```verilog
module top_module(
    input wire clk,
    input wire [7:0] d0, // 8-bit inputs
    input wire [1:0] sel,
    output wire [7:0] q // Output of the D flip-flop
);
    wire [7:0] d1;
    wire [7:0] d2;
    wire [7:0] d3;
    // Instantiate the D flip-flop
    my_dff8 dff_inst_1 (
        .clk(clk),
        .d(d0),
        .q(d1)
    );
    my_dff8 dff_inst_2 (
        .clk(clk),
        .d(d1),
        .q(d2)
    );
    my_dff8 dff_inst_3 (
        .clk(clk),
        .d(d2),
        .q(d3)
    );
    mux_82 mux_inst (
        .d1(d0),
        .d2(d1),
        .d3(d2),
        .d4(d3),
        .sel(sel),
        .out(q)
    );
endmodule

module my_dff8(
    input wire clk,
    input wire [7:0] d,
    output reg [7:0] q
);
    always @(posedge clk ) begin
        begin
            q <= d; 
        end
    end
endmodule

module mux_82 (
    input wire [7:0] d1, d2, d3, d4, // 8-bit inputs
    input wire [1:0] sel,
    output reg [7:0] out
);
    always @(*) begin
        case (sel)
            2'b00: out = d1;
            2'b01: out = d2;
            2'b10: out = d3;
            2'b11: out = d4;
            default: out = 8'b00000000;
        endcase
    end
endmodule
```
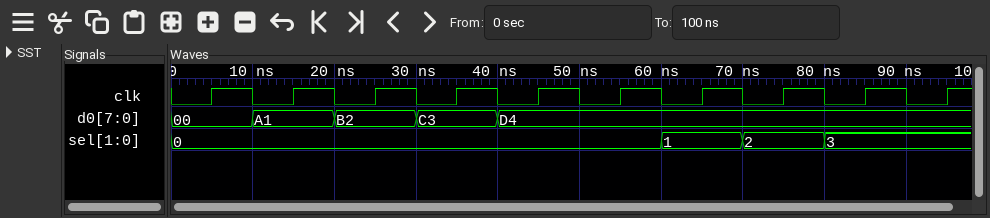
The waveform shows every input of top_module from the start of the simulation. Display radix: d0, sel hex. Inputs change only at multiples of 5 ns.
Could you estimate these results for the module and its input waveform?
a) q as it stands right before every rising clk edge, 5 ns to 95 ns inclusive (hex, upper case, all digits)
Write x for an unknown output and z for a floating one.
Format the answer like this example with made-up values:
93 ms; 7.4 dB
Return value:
00, A1, B2, C3, D4, D4, D4, D4, D4, D4
